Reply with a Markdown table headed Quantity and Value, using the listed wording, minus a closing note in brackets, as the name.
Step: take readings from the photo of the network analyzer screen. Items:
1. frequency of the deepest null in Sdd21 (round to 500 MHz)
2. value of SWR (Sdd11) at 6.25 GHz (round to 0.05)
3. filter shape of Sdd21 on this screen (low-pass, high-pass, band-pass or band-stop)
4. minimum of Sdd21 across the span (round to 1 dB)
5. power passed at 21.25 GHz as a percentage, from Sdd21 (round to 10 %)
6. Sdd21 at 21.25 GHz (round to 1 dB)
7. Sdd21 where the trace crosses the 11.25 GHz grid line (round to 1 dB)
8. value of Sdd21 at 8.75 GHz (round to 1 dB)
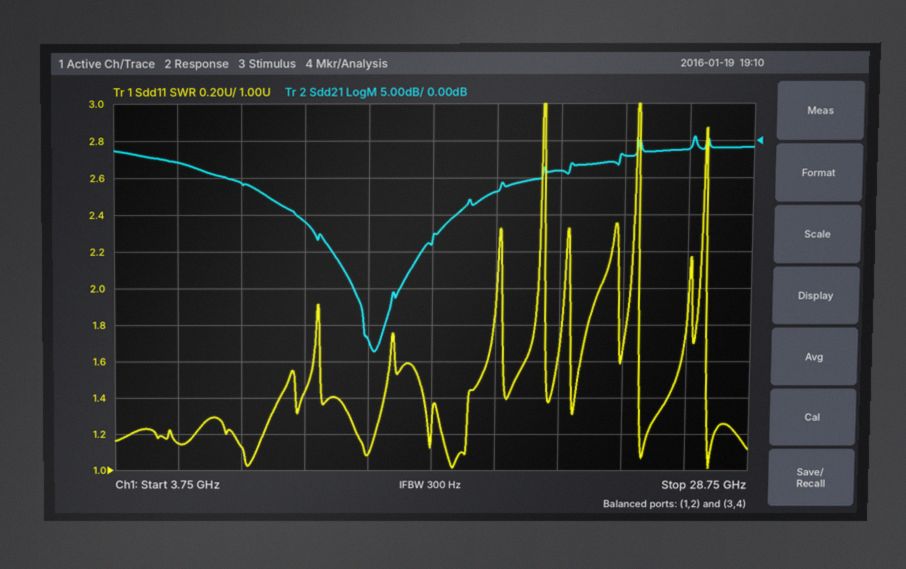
| Quantity | Value |
|---|---|
| frequency of the deepest null in Sdd21 | 14.0 GHz |
| value of SWR (Sdd11) at 6.25 GHz | 1.15 |
| filter shape of Sdd21 on this screen | band-stop |
| minimum of Sdd21 across the span | -29 dB |
| power passed at 21.25 GHz as a percentage, from Sdd21 | 40 % |
| Sdd21 at 21.25 GHz | -4 dB |
| Sdd21 where the trace crosses the 11.25 GHz grid line | -11 dB |
| value of Sdd21 at 8.75 GHz | -6 dB |
